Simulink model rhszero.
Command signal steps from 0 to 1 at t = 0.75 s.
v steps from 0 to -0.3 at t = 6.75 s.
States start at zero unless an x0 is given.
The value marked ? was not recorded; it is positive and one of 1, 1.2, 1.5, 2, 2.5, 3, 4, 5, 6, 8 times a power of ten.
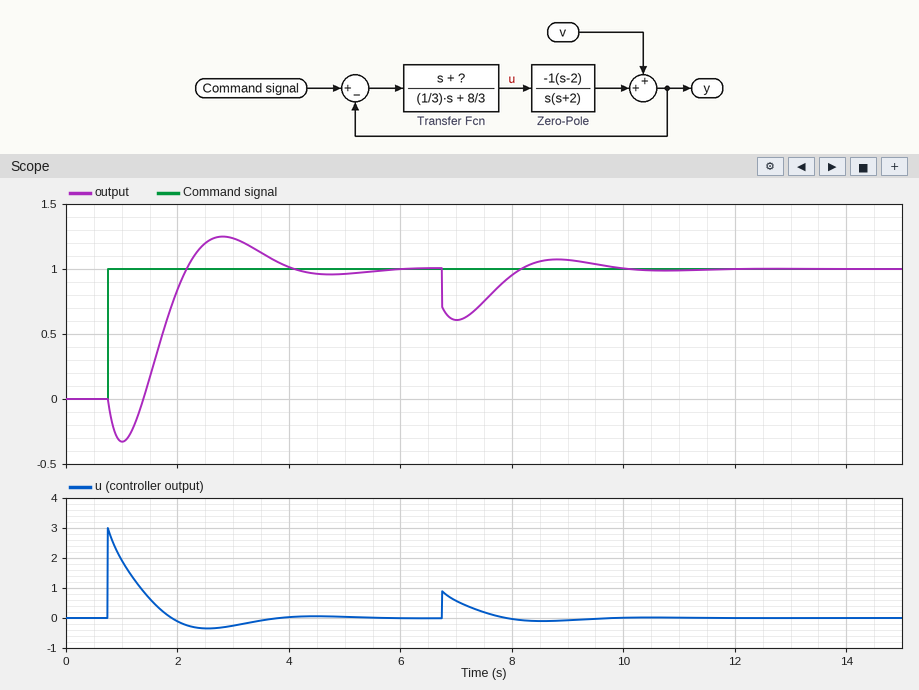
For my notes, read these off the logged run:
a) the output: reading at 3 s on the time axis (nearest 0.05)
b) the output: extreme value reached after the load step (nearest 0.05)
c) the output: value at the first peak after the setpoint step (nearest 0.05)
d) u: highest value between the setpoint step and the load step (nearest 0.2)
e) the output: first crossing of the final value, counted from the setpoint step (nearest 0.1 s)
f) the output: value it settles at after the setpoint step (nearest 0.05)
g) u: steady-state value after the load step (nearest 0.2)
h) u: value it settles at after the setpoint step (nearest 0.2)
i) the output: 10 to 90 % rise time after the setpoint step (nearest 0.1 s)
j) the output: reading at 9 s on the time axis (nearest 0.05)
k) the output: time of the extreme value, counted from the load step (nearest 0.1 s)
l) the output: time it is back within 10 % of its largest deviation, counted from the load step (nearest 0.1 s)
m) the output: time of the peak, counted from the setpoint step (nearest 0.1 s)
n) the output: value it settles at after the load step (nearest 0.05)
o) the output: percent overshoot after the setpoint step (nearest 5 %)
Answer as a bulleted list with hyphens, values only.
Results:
- 1.25
- 0.60
- 1.25
- 3.0
- 1.4 s
- 1.00
- 0.0
- 0.0
- 0.6 s
- 1.05
- 0.3 s
- 2.7 s
- 2.1 s
- 1.00
- 25 %
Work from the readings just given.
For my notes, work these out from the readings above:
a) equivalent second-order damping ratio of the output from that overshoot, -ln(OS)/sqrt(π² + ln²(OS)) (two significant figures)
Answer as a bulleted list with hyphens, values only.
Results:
- 0.40
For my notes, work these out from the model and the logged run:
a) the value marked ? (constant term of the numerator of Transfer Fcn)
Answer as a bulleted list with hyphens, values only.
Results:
- 3
